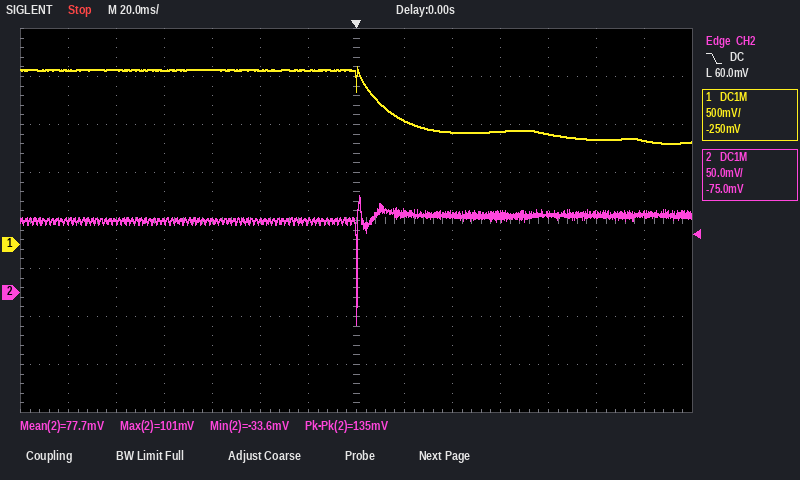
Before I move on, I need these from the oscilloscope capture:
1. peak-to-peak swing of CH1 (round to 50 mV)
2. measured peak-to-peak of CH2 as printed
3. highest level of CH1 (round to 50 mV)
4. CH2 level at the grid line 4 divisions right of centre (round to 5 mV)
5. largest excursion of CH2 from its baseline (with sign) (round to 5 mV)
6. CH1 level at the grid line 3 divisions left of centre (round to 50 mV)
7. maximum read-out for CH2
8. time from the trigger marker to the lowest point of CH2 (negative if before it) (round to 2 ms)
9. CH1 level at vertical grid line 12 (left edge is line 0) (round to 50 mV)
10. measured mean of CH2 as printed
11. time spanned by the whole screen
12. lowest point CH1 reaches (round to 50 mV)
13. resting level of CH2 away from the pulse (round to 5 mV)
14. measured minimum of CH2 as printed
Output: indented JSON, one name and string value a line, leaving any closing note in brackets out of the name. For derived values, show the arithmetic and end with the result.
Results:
{
  "peak-to-peak swing of CH1": "1.85 V − (1.05 V) = 800 mV",
  "measured peak-to-peak of CH2 as printed": "135 mV",
  "highest level of CH1": "1.85 V",
  "CH2 level at the grid line 4 divisions right of centre": "80 mV",
  "largest excursion of CH2 from its baseline (with sign)": "-110 mV",
  "CH1 level at the grid line 3 divisions left of centre": "1.80 V",
  "maximum read-out for CH2": "101 mV",
  "time from the trigger marker to the lowest point of CH2 (negative if before it)": "0 ms",
  "CH1 level at vertical grid line 12 (left edge is line 0)": "1.10 V",
  "measured mean of CH2 as printed": "77.7 mV",
  "time spanned by the whole screen": "280 ms",
  "lowest point CH1 reaches": "1.05 V",
  "resting level of CH2 away from the pulse": "75 mV",
  "measured minimum of CH2 as printed": "-33.6 mV"
}
